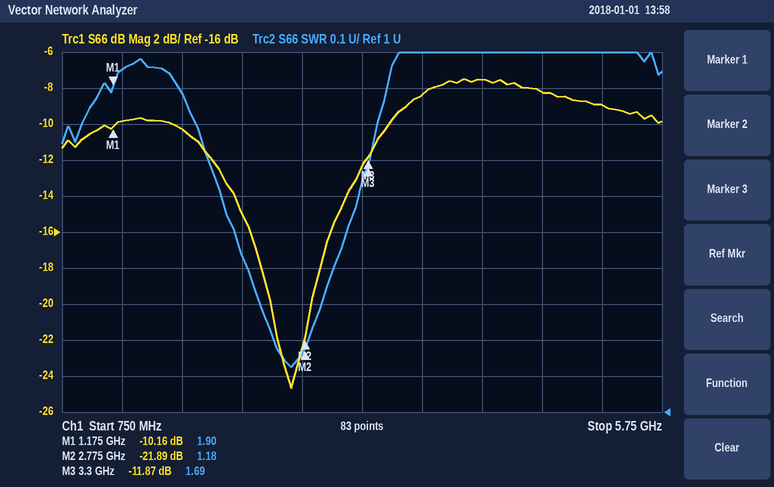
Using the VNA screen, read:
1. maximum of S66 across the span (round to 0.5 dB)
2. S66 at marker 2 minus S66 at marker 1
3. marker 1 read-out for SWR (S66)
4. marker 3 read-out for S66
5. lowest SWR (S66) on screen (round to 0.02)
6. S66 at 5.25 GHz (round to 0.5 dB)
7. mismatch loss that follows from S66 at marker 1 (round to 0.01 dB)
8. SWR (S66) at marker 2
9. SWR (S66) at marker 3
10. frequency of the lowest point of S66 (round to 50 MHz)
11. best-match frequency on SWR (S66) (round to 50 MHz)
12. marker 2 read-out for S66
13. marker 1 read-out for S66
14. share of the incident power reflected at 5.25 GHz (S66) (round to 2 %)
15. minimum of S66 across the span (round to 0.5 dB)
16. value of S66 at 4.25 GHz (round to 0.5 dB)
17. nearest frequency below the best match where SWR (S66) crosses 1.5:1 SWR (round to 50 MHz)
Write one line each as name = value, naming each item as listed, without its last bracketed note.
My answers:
maximum of S66 across the span = -7.5 dB
S66 at marker 2 minus S66 at marker 1 = -11.73 dB
marker 1 read-out for SWR = 1.90
marker 3 read-out for S66 = -11.87 dB
lowest SWR (S66) on screen = 1.12
S66 at 5.25 GHz = -9.0 dB
mismatch loss that follows from S66 at marker 1 = 0.44 dB
SWR (S66) at marker 2 = 1.18
SWR (S66) at marker 3 = 1.69
frequency of the lowest point of S66 = 2.65 GHz
best-match frequency on SWR (S66) = 2.65 GHz
marker 2 read-out for S66 = -21.89 dB
marker 1 read-out for S66 = -10.16 dB
share of the incident power reflected at 5.25 GHz (S66) = 12 %
minimum of S66 across the span = -24.5 dB
value of S66 at 4.25 GHz = -7.5 dB
nearest frequency below the best match where SWR (S66) crosses 1.5:1 SWR = 2.20 GHz
